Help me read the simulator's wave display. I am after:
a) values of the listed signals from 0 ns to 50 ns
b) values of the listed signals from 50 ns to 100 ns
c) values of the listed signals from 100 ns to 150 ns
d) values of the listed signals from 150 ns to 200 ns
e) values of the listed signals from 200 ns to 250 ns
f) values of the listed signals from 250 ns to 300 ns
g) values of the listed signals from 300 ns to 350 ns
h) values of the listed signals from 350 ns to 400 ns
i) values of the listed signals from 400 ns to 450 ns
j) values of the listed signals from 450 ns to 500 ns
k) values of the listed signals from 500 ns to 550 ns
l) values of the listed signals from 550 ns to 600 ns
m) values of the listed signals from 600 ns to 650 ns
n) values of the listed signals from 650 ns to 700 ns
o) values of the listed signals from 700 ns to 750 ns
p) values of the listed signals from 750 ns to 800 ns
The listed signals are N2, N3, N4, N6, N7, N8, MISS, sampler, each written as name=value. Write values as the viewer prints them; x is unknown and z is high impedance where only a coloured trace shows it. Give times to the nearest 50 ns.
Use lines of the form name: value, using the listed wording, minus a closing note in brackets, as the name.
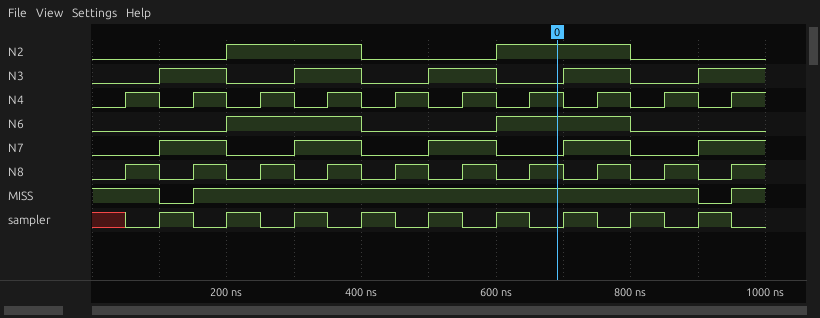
values of the listed signals from 0 ns to 50 ns: N2=0, N3=0, N4=0, N6=0, N7=0, N8=0, MISS=1, sampler=x
values of the listed signals from 50 ns to 100 ns: N2=0, N3=0, N4=1, N6=0, N7=0, N8=1, MISS=1, sampler=0
values of the listed signals from 100 ns to 150 ns: N2=0, N3=1, N4=0, N6=0, N7=1, N8=0, MISS=0, sampler=1
values of the listed signals from 150 ns to 200 ns: N2=0, N3=1, N4=1, N6=0, N7=1, N8=1, MISS=1, sampler=0
values of the listed signals from 200 ns to 250 ns: N2=1, N3=0, N4=0, N6=1, N7=0, N8=0, MISS=1, sampler=1
values of the listed signals from 250 ns to 300 ns: N2=1, N3=0, N4=1, N6=1, N7=0, N8=1, MISS=1, sampler=0
values of the listed signals from 300 ns to 350 ns: N2=1, N3=1, N4=0, N6=1, N7=1, N8=0, MISS=1, sampler=1
values of the listed signals from 350 ns to 400 ns: N2=1, N3=1, N4=1, N6=1, N7=1, N8=1, MISS=1, sampler=0
values of the listed signals from 400 ns to 450 ns: N2=0, N3=0, N4=0, N6=0, N7=0, N8=0, MISS=1, sampler=1
values of the listed signals from 450 ns to 500 ns: N2=0, N3=0, N4=1, N6=0, N7=0, N8=1, MISS=1, sampler=0
values of the listed signals from 500 ns to 550 ns: N2=0, N3=1, N4=0, N6=0, N7=1, N8=0, MISS=1, sampler=1
values of the listed signals from 550 ns to 600 ns: N2=0, N3=1, N4=1, N6=0, N7=1, N8=1, MISS=1, sampler=0
values of the listed signals from 600 ns to 650 ns: N2=1, N3=0, N4=0, N6=1, N7=0, N8=0, MISS=1, sampler=1
values of the listed signals from 650 ns to 700 ns: N2=1, N3=0, N4=1, N6=1, N7=0, N8=1, MISS=1, sampler=0
values of the listed signals from 700 ns to 750 ns: N2=1, N3=1, N4=0, N6=1, N7=1, N8=0, MISS=1, sampler=1
values of the listed signals from 750 ns to 800 ns: N2=1, N3=1, N4=1, N6=1, N7=1, N8=1, MISS=1, sampler=0
